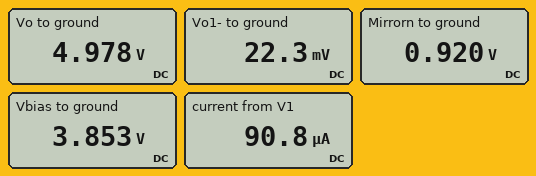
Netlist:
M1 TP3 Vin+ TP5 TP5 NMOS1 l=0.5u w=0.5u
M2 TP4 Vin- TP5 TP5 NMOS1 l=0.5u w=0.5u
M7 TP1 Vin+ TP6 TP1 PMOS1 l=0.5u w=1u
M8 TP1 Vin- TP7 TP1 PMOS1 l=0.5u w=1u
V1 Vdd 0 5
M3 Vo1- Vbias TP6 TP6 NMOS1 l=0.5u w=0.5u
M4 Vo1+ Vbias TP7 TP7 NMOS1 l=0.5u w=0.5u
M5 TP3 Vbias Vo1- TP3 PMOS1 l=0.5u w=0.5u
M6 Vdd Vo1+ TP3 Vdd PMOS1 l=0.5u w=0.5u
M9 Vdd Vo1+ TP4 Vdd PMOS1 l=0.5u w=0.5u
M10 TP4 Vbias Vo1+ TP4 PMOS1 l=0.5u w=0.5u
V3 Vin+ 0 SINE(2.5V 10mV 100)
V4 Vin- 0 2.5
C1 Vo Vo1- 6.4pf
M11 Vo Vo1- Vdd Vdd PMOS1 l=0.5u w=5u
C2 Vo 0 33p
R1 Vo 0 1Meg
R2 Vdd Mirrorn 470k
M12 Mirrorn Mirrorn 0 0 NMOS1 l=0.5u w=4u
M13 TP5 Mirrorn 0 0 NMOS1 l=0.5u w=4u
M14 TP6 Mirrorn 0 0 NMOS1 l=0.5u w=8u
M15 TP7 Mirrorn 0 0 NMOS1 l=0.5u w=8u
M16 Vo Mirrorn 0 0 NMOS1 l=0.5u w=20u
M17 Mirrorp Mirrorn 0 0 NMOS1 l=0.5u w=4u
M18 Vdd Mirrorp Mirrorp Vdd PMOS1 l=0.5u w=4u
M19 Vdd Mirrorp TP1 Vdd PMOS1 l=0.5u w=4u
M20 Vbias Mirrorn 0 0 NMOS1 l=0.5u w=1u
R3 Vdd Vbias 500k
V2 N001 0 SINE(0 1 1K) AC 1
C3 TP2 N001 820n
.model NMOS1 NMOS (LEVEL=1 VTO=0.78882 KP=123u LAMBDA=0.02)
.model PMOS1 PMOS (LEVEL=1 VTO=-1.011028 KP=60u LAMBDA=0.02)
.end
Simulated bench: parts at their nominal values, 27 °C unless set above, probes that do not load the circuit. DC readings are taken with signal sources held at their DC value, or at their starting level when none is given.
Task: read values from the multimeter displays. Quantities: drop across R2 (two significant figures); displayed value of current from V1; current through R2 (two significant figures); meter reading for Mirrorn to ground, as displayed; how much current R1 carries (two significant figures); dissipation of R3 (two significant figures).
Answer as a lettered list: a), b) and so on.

a) 4.1 V
b) 90.8 µA
c) 8.7 µA
d) 0.920 V
e) 5.0 µA
f) 2.6 µW
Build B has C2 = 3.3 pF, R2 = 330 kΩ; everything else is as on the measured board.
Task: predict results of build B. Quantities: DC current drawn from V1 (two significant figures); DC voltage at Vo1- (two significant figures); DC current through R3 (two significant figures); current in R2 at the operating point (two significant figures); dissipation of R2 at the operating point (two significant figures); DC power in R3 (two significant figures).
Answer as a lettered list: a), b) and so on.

a) 140 µA
b) 94 mV
c) 3.2 µA
d) 12 µA
e) 50 µW
f) 5.2 µW
